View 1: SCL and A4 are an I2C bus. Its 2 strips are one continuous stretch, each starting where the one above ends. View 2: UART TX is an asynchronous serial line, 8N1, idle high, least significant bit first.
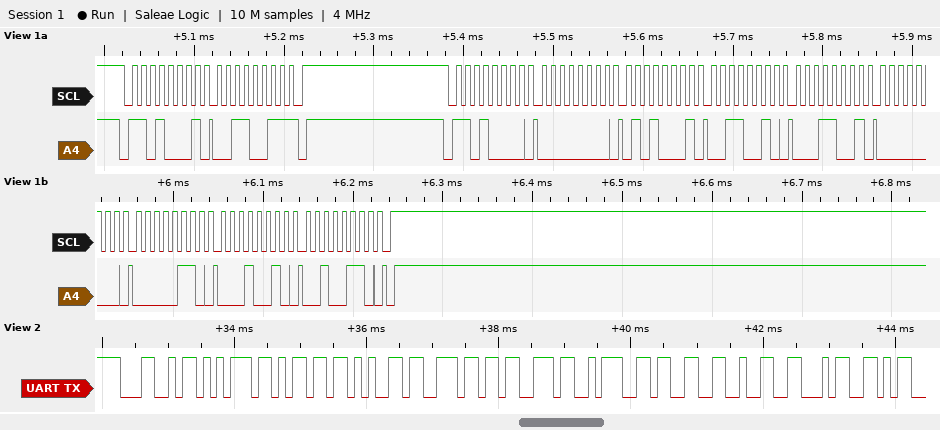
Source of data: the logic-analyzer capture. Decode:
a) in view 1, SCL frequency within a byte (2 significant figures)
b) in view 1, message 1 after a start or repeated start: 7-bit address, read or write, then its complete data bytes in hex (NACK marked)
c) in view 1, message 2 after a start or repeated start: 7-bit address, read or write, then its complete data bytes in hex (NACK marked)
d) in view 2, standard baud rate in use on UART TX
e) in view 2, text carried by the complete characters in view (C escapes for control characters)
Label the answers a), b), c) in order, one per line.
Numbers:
a) 100 kHz
b) 0x68 read: 33 NACK
c) 0x68 write: 00 51 32 19 00 06 12 26
d) 9600 baud
e) "Lumens:324"
